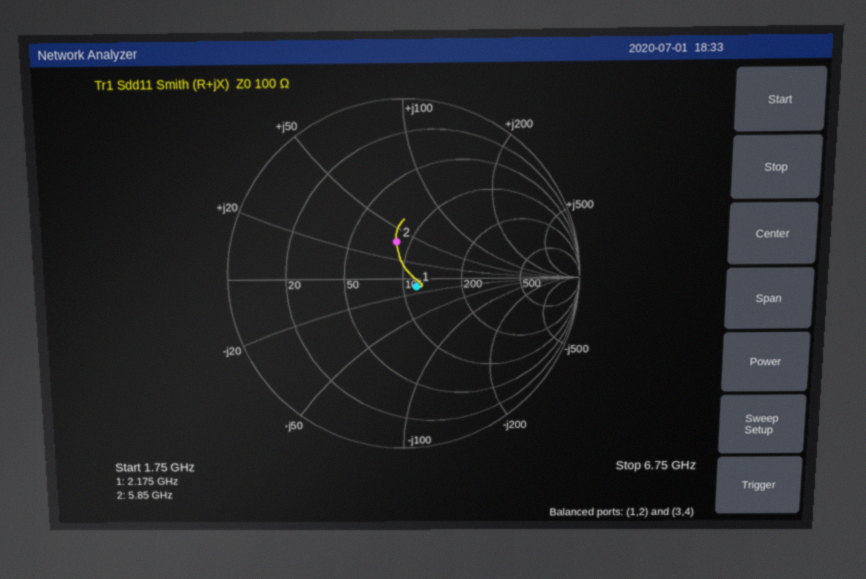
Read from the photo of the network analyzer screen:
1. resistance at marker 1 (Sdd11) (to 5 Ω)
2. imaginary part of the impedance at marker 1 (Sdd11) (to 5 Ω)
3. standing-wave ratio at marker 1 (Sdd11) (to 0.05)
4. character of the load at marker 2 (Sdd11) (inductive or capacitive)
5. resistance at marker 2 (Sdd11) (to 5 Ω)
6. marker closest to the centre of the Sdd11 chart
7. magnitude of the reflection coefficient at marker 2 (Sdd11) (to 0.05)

115 Ω
-10 Ω
1.20
inductive
85 Ω
marker 1
0.20
